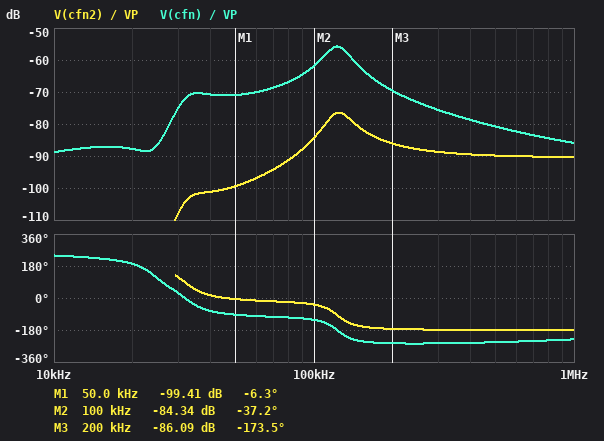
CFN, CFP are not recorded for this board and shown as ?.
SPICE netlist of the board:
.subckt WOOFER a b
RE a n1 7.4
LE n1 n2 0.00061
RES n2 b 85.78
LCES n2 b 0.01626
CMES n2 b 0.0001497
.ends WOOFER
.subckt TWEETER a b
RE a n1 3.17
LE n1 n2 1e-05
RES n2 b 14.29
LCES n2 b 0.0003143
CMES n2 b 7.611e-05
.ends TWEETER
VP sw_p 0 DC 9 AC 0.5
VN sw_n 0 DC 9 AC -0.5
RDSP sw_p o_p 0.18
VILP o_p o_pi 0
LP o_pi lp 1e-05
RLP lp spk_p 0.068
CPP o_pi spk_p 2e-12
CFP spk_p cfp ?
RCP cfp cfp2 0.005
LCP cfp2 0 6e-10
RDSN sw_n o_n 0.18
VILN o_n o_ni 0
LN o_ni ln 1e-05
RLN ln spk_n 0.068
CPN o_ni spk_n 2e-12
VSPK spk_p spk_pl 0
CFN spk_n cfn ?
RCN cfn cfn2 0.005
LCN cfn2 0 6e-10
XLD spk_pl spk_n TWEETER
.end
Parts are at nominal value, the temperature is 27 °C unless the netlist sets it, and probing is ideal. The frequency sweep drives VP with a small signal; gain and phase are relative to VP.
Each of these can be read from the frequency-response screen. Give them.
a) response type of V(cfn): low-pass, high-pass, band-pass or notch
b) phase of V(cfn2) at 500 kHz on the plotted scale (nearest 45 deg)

band-pass
-180 deg
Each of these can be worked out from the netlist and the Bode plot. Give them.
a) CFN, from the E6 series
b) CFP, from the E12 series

330 nF
3.3 µF
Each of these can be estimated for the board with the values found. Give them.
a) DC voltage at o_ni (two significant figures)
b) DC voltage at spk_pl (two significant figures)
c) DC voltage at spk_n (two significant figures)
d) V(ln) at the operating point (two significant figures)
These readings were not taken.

9.0 V
9.0 V
9.0 V
9.0 V
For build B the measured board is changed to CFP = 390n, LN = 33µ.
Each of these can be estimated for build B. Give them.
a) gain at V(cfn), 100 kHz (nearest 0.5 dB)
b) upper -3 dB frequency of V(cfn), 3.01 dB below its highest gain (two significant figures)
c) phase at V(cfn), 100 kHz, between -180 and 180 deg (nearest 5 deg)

-61.0 dB
69 kHz
-100 deg
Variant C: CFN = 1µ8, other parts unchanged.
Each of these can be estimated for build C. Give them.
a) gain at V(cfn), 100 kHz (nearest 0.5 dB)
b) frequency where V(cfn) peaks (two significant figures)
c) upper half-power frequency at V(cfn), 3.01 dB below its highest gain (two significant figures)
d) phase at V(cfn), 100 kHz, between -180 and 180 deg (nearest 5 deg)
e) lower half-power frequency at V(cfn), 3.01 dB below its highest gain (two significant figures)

-64.5 dB
32 kHz
60 kHz
105 deg
30 kHz
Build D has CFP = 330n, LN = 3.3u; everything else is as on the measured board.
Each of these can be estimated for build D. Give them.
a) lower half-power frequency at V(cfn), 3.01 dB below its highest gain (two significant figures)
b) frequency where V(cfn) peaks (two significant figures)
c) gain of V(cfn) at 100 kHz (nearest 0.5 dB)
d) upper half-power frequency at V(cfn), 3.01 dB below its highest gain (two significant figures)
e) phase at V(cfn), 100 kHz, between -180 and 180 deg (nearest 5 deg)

170 kHz
180 kHz
-68.5 dB
200 kHz
-40 deg
